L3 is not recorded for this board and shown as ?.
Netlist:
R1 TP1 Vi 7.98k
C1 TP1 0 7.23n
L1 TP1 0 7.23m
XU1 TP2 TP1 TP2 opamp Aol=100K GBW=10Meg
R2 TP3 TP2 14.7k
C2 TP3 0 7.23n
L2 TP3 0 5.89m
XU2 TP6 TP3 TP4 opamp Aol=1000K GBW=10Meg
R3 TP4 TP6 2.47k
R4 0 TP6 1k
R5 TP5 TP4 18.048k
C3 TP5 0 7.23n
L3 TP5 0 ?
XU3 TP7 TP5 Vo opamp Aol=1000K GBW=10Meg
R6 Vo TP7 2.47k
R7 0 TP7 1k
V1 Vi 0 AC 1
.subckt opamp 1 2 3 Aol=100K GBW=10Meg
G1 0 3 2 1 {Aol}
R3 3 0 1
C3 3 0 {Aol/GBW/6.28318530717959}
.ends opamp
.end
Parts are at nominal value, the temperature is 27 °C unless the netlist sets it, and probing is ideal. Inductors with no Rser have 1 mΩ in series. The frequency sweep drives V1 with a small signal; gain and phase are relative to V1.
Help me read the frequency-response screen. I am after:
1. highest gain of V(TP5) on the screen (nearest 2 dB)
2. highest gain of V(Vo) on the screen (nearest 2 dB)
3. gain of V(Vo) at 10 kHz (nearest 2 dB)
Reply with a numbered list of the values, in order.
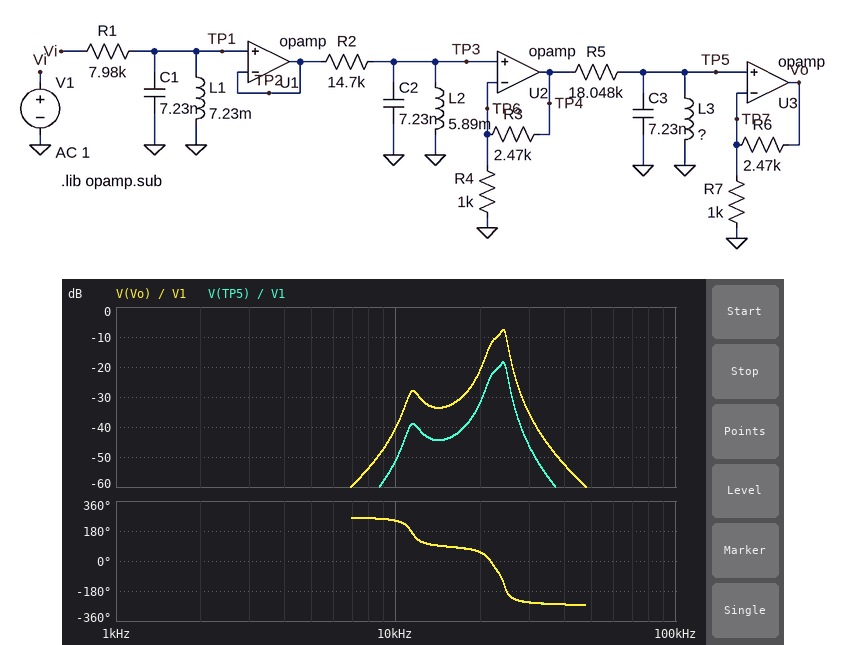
1. -18 dB
2. -8 dB
3. -40 dB
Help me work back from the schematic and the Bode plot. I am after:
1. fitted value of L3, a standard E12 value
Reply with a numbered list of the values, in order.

1. 27 mH
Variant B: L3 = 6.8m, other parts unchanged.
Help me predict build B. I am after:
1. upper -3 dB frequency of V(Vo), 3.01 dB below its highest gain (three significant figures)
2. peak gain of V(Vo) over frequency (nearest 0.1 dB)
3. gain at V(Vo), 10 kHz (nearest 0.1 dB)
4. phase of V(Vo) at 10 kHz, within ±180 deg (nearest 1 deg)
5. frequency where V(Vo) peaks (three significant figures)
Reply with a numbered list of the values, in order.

1. 23.7 kHz
2. 12.7 dB
3. -62.3 dB
4. -98 deg
5. 22.8 kHz
